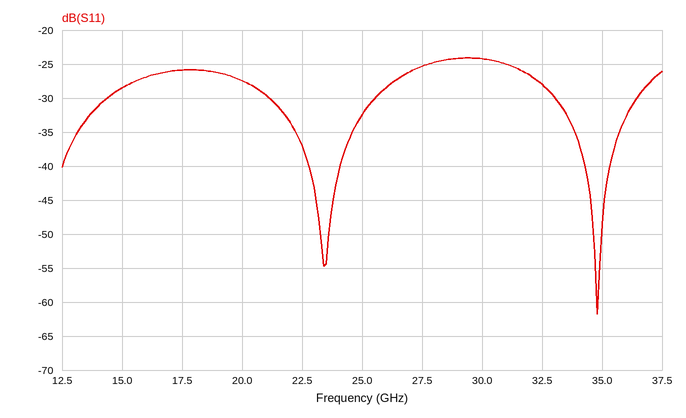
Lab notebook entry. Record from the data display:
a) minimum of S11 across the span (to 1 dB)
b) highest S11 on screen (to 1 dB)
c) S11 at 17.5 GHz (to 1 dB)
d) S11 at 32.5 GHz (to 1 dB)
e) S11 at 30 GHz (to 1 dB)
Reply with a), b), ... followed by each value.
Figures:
a) -62 dB
b) -24 dB
c) -26 dB
d) -28 dB
e) -24 dB
